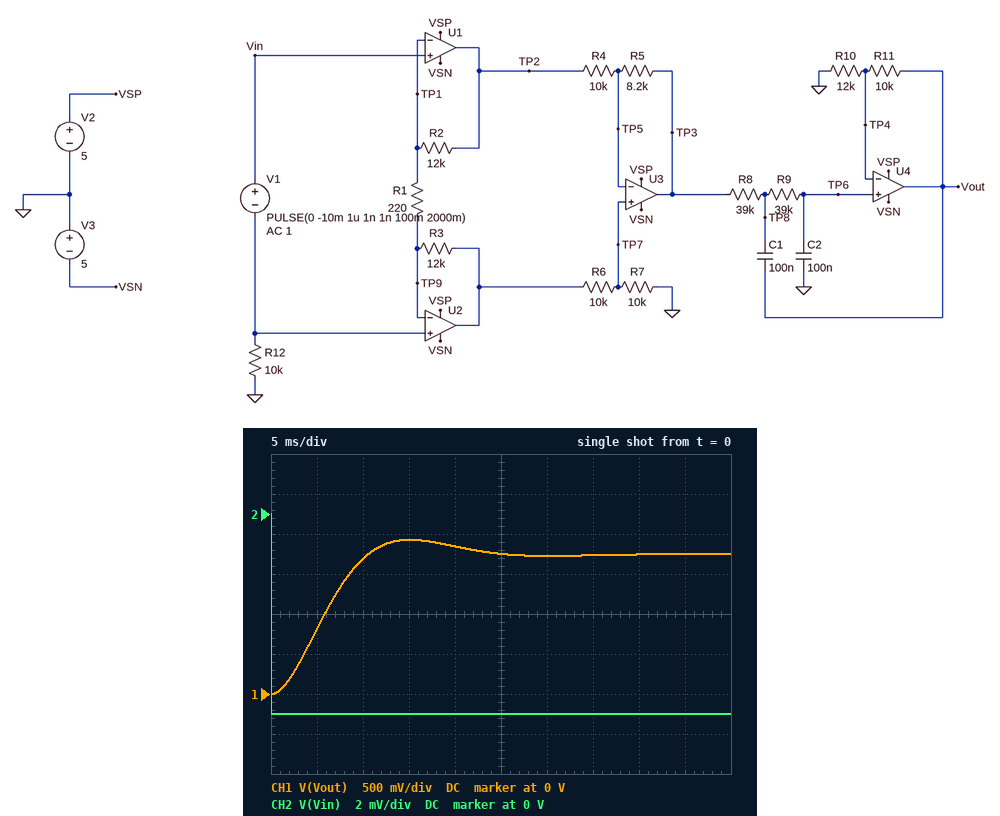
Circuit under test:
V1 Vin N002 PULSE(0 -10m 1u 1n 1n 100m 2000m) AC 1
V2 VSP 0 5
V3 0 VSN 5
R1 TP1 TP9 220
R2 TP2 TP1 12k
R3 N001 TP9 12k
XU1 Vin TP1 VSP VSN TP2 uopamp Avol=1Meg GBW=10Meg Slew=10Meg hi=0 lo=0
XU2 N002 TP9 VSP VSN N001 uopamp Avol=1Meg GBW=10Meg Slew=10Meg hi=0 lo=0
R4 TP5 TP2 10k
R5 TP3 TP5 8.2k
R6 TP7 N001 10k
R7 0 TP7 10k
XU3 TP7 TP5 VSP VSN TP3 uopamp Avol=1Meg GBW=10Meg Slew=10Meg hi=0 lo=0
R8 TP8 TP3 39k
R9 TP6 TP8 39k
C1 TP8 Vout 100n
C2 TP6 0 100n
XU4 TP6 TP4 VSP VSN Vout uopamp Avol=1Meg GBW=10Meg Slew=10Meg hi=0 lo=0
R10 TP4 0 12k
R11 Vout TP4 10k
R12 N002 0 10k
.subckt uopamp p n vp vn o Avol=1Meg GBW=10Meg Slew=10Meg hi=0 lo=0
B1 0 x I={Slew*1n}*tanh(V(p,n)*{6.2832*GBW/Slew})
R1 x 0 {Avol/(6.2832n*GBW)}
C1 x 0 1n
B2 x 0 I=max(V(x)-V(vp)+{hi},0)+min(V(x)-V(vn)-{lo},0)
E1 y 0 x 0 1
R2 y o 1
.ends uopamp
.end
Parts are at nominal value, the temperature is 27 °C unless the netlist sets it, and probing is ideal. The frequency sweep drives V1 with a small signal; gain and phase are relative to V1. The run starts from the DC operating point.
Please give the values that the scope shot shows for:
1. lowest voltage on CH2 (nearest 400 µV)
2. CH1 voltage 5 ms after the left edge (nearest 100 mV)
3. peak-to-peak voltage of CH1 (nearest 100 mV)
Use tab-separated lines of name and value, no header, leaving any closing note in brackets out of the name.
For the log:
lowest voltage on CH2	-10.0 mV
CH1 voltage 5 ms after the left edge	800 mV
peak-to-peak voltage of CH1	1.9 V
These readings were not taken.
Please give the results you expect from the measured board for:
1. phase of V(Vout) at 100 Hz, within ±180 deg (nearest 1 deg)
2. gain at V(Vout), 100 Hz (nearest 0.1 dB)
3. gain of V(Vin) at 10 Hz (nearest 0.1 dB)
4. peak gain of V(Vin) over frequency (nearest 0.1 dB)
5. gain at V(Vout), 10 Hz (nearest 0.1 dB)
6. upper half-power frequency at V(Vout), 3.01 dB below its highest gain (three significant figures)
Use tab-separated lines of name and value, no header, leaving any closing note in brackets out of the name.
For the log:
phase of V(Vout) at 100 Hz, within ±180 deg	30 deg
gain at V(Vout), 100 Hz	29.6 dB
gain of V(Vin) at 10 Hz	0 dB
peak gain of V(Vin) over frequency	0 dB
gain at V(Vout), 10 Hz	45.0 dB
upper half-power frequency at V(Vout), 3.01 dB below its highest gain	45.9 Hz
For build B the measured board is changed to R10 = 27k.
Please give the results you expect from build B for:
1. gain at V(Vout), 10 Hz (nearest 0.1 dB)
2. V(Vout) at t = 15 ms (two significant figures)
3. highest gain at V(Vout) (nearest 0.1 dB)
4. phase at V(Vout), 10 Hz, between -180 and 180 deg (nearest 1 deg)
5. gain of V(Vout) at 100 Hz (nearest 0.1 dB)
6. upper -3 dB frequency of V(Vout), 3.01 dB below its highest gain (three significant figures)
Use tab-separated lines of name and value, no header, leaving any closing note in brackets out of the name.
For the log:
gain at V(Vout), 10 Hz	42.1 dB
V(Vout) at t = 15 ms	1.3 V
highest gain at V(Vout)	42.3 dB
phase at V(Vout), 10 Hz, between -180 and 180 deg	157 deg
gain of V(Vout) at 100 Hz	26.2 dB
upper -3 dB frequency of V(Vout), 3.01 dB below its highest gain	34.7 Hz
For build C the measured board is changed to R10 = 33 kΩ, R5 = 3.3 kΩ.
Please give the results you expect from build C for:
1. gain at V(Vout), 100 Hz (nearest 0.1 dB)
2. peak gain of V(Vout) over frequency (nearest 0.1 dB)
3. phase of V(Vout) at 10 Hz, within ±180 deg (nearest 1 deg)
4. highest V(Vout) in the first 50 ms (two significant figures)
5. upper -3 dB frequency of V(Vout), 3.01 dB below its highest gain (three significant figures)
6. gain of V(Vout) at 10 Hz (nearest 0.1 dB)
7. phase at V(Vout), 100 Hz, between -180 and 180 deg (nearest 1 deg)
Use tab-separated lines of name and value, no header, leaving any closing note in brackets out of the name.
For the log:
gain at V(Vout), 100 Hz	20.8 dB
peak gain of V(Vout) over frequency	37.0 dB
phase of V(Vout) at 10 Hz, within ±180 deg	156 deg
highest V(Vout) in the first 50 ms	720 mV
upper -3 dB frequency of V(Vout), 3.01 dB below its highest gain	33.0 Hz
gain of V(Vout) at 10 Hz	36.8 dB
phase at V(Vout), 100 Hz, between -180 and 180 deg	40 deg
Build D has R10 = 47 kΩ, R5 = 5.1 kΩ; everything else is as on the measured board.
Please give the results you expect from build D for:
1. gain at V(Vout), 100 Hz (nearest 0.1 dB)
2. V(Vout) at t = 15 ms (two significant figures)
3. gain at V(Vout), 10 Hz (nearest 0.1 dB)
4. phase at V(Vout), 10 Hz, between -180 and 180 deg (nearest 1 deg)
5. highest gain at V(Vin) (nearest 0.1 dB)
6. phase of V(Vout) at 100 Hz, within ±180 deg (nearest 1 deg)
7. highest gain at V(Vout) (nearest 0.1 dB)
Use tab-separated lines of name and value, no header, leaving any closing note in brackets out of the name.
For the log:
gain at V(Vout), 100 Hz	22.1 dB
V(Vout) at t = 15 ms	790 mV
gain at V(Vout), 10 Hz	38.2 dB
phase at V(Vout), 10 Hz, between -180 and 180 deg	155 deg
highest gain at V(Vin)	0 dB
phase of V(Vout) at 100 Hz, within ±180 deg	41 deg
highest gain at V(Vout)	38.5 dB
